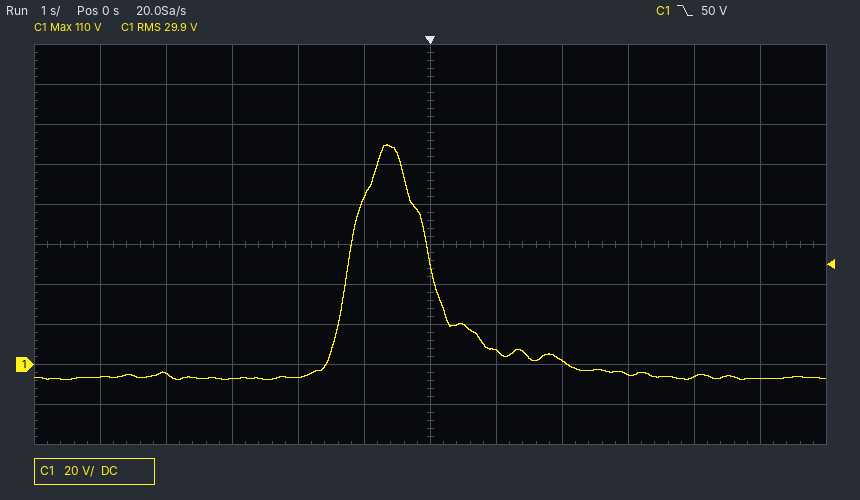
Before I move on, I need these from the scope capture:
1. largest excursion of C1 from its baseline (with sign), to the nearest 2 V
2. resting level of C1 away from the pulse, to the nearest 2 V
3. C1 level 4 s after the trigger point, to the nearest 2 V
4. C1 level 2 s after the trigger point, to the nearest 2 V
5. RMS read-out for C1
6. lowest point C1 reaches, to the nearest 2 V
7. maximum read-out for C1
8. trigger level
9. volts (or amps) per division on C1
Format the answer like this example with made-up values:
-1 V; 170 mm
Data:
+116 V; -6 V; -6 V; 2 V; 29.9 V; -8 V; 110 V; 50 V; 20 V
